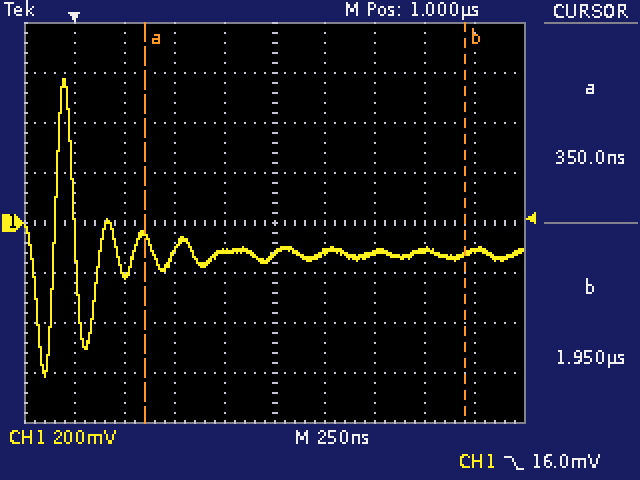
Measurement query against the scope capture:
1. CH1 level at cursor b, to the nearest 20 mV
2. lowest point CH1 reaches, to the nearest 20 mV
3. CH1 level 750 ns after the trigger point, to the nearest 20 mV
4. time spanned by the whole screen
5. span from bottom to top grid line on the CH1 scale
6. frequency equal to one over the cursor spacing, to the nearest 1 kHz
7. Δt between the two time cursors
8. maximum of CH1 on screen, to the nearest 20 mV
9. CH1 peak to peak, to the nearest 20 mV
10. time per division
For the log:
-120 mV
-620 mV
-120 mV
2.5 µs
1.6 V
625 kHz
1.600 µs
580 mV
1.20 V
250 ns
